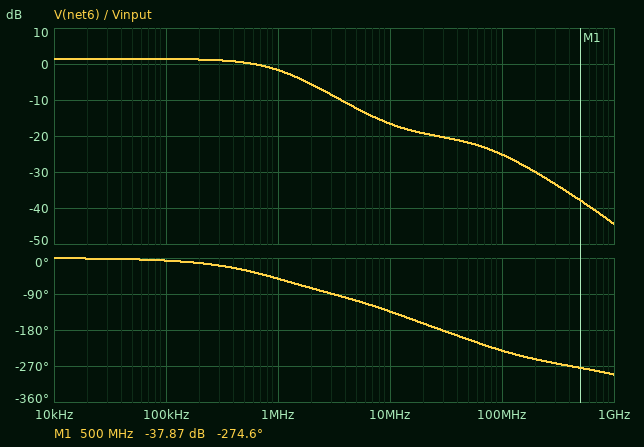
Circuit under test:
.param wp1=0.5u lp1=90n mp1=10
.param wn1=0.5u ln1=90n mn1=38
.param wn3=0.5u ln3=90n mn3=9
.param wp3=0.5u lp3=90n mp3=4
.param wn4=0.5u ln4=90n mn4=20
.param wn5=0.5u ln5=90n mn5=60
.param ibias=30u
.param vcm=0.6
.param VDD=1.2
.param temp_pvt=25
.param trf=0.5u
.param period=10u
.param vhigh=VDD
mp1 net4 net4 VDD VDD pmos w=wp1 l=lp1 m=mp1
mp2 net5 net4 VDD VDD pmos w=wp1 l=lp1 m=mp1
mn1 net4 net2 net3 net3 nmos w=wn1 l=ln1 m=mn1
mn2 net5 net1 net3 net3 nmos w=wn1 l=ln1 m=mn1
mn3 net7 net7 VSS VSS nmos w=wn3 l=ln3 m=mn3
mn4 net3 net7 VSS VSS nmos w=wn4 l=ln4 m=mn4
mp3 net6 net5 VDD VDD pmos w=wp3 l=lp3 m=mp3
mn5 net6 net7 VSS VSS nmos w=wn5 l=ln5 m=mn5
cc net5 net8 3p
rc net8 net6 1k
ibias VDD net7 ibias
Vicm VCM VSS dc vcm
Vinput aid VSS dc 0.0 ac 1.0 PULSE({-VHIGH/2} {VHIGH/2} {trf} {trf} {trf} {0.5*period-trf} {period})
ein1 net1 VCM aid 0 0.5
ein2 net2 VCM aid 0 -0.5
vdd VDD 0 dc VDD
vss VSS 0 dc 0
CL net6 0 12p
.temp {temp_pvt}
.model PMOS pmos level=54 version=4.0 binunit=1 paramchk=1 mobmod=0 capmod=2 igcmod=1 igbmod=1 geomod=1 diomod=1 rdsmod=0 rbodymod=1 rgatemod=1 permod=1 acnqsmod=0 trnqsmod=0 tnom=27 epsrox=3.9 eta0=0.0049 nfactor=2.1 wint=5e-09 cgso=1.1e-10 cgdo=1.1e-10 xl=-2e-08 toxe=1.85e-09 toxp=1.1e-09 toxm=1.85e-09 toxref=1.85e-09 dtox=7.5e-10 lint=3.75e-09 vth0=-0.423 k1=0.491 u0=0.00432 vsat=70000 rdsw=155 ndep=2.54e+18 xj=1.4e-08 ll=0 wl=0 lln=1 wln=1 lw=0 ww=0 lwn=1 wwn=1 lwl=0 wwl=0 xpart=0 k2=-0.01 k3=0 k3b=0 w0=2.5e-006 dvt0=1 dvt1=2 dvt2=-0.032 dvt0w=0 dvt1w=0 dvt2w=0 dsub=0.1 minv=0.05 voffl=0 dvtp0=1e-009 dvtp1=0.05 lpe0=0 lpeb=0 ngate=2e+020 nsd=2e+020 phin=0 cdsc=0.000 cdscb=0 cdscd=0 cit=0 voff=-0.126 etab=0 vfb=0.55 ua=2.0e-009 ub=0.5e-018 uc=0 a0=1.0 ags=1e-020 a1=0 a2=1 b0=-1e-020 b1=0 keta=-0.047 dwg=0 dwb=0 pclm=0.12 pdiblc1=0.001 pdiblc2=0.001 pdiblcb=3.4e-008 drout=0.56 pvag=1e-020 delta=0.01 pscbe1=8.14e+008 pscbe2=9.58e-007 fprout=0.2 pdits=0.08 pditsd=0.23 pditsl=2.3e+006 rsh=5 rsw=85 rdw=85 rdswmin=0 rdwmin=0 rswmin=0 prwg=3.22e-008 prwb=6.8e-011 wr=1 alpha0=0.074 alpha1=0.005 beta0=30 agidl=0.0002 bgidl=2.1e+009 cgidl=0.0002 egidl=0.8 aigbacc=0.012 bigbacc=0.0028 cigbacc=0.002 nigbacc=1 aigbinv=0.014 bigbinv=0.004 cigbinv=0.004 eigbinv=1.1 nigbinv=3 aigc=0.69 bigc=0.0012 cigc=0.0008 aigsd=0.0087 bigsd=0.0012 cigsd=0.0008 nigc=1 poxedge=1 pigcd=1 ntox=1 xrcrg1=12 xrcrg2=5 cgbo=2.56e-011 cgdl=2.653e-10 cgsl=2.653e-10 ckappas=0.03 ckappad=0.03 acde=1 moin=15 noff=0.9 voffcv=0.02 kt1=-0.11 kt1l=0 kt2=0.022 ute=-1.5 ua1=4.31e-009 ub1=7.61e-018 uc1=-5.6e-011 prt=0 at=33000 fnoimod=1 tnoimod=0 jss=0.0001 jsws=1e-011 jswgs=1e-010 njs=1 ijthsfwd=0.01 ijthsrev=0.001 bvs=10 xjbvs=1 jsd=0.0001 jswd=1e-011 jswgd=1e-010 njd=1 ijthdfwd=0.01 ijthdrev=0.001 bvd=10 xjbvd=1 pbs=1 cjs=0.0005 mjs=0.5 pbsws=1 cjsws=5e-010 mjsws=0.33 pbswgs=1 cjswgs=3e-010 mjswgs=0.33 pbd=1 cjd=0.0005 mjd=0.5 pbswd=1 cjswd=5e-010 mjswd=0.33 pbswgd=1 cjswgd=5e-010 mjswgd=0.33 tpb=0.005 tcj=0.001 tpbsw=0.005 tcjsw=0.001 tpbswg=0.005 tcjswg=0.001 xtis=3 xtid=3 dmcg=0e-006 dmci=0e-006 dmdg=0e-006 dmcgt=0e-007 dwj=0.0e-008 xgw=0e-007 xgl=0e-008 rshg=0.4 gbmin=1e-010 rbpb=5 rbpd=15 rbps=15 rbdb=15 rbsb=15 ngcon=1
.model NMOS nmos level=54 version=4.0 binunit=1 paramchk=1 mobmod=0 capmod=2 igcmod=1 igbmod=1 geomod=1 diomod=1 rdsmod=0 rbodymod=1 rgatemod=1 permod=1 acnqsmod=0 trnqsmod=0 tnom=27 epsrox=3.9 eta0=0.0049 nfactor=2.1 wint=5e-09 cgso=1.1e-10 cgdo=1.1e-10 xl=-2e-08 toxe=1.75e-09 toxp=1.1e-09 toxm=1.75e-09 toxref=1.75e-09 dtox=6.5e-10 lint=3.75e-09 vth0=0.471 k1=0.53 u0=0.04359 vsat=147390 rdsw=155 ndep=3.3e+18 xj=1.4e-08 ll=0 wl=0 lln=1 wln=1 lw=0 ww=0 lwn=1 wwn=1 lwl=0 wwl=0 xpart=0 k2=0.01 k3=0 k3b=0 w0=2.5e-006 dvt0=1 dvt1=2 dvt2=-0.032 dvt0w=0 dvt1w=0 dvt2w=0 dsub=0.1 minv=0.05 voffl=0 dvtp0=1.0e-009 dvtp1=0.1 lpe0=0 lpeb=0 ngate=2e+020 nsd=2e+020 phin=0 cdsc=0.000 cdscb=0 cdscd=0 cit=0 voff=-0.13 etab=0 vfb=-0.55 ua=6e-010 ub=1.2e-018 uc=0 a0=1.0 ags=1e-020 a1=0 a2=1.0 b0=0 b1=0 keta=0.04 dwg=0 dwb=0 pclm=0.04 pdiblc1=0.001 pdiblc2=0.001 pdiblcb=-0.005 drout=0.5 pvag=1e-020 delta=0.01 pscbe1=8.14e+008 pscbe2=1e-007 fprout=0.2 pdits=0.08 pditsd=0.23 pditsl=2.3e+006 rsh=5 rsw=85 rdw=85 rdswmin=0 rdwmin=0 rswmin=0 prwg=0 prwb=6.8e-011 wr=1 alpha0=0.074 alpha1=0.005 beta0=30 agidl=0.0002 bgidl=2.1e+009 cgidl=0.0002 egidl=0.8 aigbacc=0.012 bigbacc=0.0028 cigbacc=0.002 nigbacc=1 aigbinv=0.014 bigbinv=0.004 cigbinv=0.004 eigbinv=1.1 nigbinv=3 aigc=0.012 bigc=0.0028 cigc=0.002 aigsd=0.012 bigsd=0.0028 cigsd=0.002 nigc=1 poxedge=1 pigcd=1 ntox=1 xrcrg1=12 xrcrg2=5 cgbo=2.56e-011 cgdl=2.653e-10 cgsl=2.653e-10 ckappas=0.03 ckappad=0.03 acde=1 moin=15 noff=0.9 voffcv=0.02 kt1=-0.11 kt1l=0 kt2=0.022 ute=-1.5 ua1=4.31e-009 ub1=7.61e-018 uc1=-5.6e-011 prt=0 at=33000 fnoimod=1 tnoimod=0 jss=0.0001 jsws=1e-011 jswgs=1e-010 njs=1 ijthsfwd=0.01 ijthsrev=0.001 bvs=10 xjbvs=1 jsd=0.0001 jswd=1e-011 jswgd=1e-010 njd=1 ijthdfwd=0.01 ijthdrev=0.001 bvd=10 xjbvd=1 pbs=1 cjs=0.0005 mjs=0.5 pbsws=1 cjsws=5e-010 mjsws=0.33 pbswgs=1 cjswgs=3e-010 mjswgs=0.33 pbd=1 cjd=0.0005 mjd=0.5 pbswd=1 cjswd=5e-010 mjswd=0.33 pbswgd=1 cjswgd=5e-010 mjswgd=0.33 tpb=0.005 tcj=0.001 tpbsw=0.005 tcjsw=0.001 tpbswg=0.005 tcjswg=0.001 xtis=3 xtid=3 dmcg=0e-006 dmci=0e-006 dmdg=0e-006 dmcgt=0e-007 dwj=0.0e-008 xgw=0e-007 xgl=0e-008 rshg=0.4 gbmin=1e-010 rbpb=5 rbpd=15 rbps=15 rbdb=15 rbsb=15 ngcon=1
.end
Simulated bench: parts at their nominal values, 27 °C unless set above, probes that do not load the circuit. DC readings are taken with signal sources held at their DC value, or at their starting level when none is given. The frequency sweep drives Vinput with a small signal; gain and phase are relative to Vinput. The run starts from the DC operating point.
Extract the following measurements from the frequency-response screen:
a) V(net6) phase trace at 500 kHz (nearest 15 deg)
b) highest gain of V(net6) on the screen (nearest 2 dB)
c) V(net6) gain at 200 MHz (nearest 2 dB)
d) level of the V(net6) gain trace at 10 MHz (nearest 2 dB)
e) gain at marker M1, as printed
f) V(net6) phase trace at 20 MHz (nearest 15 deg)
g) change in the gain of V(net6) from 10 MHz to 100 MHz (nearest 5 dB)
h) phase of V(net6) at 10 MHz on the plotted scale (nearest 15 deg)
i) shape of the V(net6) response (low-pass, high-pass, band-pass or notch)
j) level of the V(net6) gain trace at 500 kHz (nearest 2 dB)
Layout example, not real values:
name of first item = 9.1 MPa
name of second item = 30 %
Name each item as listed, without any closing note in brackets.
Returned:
V(net6) phase trace at 500 kHz = -30 deg
highest gain of V(net6) on the screen = 2 dB
V(net6) gain at 200 MHz = -30 dB
level of the V(net6) gain trace at 10 MHz = -16 dB
gain at marker M1, as printed = -37.87 dB
V(net6) phase trace at 20 MHz = -165 deg
change in the gain of V(net6) from 10 MHz to 100 MHz = -10 dB
phase of V(net6) at 10 MHz on the plotted scale = -135 deg
shape of the V(net6) response = low-pass
level of the V(net6) gain trace at 500 kHz = 0 dB
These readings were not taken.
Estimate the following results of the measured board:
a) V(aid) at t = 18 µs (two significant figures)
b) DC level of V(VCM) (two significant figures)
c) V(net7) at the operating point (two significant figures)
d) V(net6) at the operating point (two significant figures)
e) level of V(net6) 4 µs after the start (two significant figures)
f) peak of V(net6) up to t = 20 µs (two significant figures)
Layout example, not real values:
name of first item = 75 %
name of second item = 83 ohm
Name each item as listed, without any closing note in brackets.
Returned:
V(aid) at t = 18 µs = -600 mV
DC level of V(VCM) = 600 mV
V(net7) at the operating point = 430 mV
V(net6) at the operating point = 3.0 mV
level of V(net6) 4 µs after the start = 820 mV
peak of V(net6) up to t = 20 µs = 820 mV
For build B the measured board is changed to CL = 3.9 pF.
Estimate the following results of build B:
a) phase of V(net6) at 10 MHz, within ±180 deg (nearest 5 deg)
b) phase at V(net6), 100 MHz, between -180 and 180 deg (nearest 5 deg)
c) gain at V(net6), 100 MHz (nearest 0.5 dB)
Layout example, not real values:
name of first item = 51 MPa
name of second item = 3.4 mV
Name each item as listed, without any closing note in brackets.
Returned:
phase of V(net6) at 10 MHz, within ±180 deg = -130 deg
phase at V(net6), 100 MHz, between -180 and 180 deg = 160 deg
gain at V(net6), 100 MHz = -21.0 dB
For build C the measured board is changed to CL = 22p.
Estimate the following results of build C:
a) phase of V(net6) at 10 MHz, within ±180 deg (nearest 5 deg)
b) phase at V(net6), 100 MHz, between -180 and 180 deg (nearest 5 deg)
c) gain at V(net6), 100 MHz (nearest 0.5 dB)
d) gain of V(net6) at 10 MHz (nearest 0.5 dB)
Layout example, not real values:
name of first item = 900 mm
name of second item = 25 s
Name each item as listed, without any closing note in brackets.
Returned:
phase of V(net6) at 10 MHz, within ±180 deg = -140 deg
phase at V(net6), 100 MHz, between -180 and 180 deg = 115 deg
gain at V(net6), 100 MHz = -29.5 dB
gain of V(net6) at 10 MHz = -17.0 dB
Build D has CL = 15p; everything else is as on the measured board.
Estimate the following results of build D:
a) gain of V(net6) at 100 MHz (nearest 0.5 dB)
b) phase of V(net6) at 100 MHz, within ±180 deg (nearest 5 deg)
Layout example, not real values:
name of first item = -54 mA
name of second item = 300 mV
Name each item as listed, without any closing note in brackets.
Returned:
gain of V(net6) at 100 MHz = -26.5 dB
phase of V(net6) at 100 MHz, within ±180 deg = 125 deg
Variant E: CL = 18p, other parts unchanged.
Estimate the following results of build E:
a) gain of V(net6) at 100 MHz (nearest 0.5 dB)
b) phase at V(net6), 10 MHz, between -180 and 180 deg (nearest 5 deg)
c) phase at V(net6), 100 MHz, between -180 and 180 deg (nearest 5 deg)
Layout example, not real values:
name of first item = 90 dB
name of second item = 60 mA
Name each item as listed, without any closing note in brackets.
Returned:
gain of V(net6) at 100 MHz = -28.0 dB
phase at V(net6), 10 MHz, between -180 and 180 deg = -140 deg
phase at V(net6), 100 MHz, between -180 and 180 deg = 120 deg
